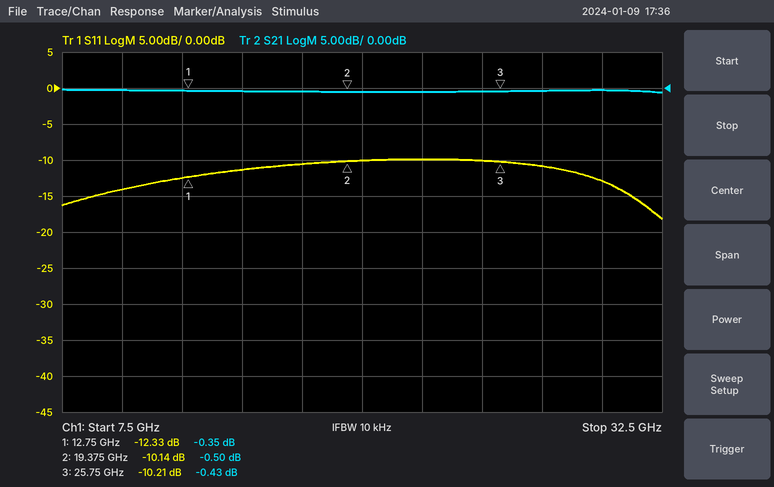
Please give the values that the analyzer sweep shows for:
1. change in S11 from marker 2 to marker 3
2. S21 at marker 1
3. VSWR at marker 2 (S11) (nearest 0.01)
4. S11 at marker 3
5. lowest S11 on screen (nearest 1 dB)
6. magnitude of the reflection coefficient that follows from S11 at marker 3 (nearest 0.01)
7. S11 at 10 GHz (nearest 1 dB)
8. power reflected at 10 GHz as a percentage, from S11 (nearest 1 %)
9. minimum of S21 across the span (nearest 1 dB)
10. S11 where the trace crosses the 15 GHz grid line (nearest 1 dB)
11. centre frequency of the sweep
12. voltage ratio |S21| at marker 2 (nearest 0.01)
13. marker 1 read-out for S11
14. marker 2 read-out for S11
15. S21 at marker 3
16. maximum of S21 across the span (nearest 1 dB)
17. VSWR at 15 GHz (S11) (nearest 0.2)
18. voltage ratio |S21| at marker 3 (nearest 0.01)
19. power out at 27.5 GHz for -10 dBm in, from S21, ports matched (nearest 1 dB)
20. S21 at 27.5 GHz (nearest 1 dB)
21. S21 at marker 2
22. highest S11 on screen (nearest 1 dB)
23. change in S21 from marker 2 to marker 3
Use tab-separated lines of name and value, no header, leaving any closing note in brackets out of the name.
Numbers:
change in S11 from marker 2 to marker 3	-0.07 dB
S21 at marker 1	-0.35 dB
VSWR at marker 2 (S11)	1.90
S11 at marker 3	-10.21 dB
lowest S11 on screen	-18 dB
magnitude of the reflection coefficient that follows from S11 at marker 3	0.31
S11 at 10 GHz	-14 dB
power reflected at 10 GHz as a percentage, from S11	4 %
minimum of S21 across the span	-1 dB
S11 where the trace crosses the 15 GHz grid line	-11 dB
centre frequency of the sweep	20 GHz
voltage ratio |S21| at marker 2	0.94
marker 1 read-out for S11	-12.33 dB
marker 2 read-out for S11	-10.14 dB
S21 at marker 3	-0.43 dB
maximum of S21 across the span	0 dB
VSWR at 15 GHz (S11)	1.8
voltage ratio |S21| at marker 3	0.95
power out at 27.5 GHz for -10 dBm in, from S21, ports matched	-10 dBm
S21 at 27.5 GHz	0 dB
S21 at marker 2	-0.50 dB
highest S11 on screen	-10 dB
change in S21 from marker 2 to marker 3	0.07 dB
